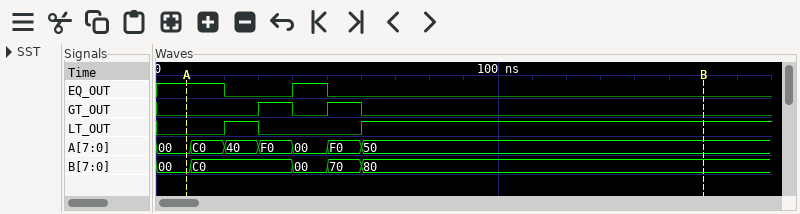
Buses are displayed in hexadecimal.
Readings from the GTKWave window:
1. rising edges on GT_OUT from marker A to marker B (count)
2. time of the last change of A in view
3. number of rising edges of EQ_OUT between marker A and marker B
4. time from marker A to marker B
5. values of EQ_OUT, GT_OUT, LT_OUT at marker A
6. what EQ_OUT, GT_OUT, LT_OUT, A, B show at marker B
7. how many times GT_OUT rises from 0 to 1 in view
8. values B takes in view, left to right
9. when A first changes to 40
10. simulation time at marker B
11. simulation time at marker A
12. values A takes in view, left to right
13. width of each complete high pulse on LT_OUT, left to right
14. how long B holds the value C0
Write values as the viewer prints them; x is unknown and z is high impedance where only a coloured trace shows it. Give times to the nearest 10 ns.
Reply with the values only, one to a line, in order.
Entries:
2
60 ns
1
150 ns
EQ_OUT=1, GT_OUT=0, LT_OUT=0
EQ_OUT=0, GT_OUT=0, LT_OUT=1, A=50, B=80
2
00, C0, 00, 70, 80
20 ns
160 ns
10 ns
00, C0, 40, F0, 00, F0, 50
10 ns
30 ns
